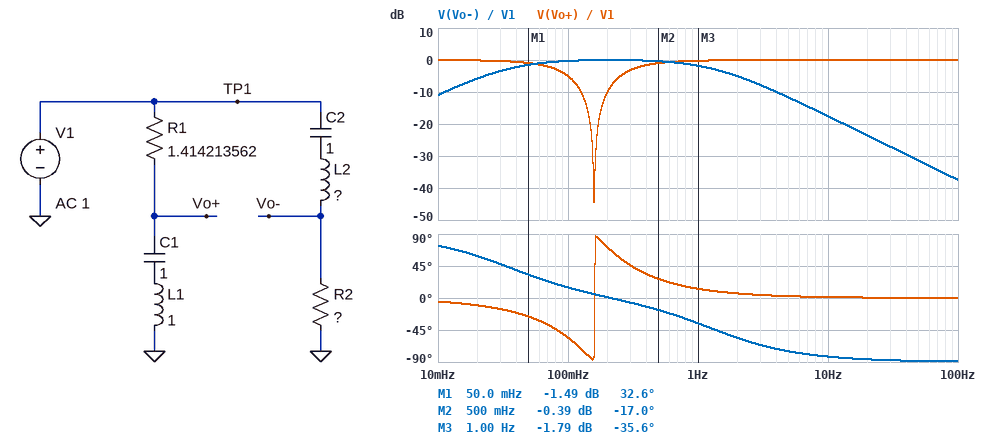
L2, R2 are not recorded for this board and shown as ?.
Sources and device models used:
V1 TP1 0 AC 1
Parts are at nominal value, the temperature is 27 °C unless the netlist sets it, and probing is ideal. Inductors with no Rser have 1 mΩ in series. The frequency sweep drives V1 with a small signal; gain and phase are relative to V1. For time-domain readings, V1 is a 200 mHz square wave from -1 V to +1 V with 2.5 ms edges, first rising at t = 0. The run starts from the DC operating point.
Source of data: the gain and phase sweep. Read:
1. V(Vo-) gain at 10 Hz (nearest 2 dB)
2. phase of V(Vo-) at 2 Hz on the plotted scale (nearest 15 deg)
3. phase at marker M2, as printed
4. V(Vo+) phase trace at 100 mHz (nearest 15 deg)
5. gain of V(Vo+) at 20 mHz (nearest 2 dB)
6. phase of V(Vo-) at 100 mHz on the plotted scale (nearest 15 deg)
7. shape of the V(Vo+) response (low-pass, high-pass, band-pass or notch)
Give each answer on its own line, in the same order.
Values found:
-18 dB
-60 deg
-17.0 deg
-60 deg
0 dB
15 deg
notch
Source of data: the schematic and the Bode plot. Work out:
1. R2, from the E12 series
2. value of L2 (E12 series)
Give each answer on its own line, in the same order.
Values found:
4.7 Ω
560 mH
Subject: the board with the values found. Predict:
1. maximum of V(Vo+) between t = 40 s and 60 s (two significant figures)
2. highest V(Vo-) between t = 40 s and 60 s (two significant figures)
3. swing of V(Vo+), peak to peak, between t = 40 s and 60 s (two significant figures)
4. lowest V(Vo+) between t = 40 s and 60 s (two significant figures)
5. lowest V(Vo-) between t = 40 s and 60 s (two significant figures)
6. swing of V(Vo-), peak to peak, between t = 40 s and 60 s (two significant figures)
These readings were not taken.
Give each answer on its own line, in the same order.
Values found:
1.7 V
1.2 V
3.4 V
-1.7 V
-1.2 V
2.3 V
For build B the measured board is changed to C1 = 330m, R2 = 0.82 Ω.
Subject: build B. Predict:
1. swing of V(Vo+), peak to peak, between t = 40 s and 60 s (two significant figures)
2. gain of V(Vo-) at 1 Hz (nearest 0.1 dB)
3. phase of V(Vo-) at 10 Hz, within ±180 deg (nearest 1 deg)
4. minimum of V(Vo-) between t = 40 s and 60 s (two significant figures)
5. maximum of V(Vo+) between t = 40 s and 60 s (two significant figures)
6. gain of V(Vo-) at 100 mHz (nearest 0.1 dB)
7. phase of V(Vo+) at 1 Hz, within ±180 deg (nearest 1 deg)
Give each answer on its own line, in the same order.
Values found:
2.6 V
-12.5 dB
-89 deg
-1.3 V
1.3 V
-5.2 dB
14 deg
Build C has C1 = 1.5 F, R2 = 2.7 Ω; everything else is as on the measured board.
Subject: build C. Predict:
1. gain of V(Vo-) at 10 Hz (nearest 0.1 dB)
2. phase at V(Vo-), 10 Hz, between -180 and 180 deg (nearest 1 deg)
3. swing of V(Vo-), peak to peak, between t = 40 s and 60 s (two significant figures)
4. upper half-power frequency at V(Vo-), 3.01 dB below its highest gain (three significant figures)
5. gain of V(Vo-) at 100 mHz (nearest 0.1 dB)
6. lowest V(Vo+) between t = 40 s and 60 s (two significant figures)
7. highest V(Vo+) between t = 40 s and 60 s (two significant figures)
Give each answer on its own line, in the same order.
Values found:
-22.3 dB
-86 deg
2.4 V
823 mHz
-0.8 dB
-1.8 V
1.8 V
